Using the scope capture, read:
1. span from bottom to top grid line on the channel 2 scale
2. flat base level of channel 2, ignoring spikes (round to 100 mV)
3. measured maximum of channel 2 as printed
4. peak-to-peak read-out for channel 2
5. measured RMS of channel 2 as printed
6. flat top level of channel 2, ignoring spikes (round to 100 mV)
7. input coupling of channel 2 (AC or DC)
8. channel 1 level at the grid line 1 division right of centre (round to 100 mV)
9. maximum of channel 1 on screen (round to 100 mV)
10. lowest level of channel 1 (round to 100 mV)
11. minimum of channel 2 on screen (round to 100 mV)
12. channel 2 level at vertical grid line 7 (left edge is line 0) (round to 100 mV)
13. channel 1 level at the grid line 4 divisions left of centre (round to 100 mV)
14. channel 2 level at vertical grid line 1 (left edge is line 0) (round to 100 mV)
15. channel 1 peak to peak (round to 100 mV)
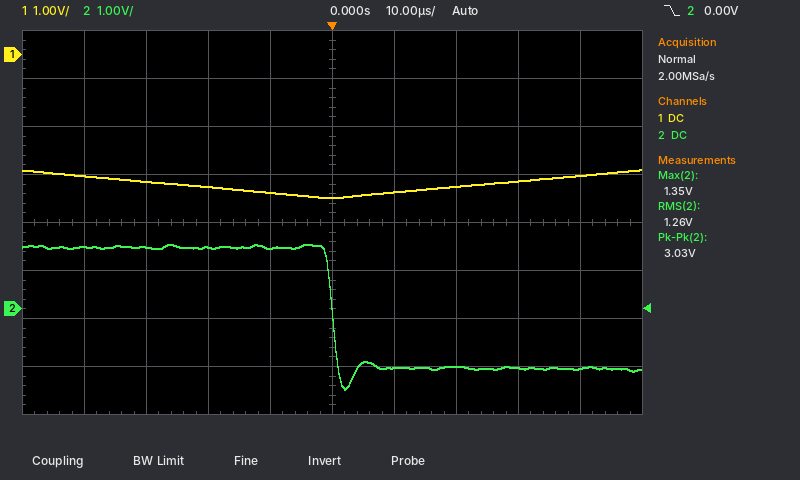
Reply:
8 V
-1.2 V
1.35 V
3.03 V
1.26 V
1.3 V
DC
-2.9 V
-2.4 V
-3.0 V
-1.7 V
-1.2 V
-2.5 V
1.3 V
600 mV
